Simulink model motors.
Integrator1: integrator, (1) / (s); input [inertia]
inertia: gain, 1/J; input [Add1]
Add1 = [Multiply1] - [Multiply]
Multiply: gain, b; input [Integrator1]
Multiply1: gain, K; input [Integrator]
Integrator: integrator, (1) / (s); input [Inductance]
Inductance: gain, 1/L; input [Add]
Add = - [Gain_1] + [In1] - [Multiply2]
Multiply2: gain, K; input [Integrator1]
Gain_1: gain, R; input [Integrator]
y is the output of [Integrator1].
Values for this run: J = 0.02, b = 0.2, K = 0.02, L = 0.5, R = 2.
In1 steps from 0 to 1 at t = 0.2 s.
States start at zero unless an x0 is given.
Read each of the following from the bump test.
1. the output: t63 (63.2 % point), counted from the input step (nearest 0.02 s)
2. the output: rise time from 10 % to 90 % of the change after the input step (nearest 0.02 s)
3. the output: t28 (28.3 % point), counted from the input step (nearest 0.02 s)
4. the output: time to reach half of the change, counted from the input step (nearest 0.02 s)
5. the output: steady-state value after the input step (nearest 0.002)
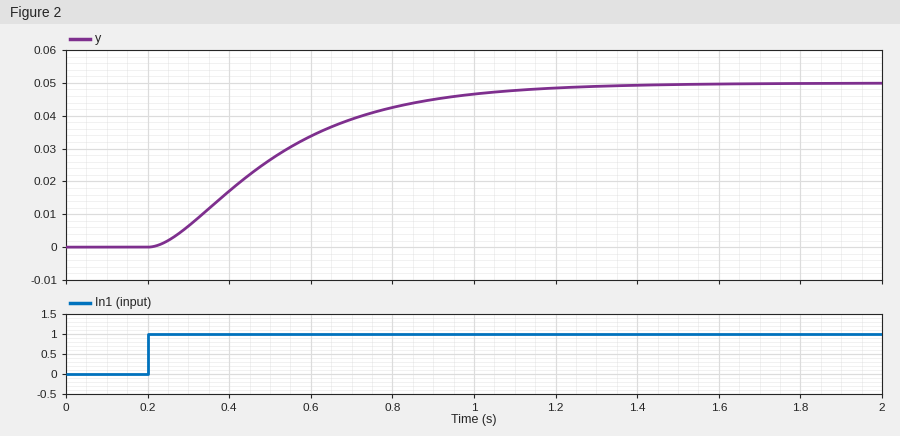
0.36 s
0.62 s
0.18 s
0.28 s
0.050
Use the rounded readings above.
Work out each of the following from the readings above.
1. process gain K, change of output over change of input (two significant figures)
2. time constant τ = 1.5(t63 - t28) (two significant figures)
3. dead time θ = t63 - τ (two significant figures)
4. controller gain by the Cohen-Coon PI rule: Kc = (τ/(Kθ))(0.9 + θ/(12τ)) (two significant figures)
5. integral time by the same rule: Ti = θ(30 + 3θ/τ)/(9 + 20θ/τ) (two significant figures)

0.050
0.27 s
0.090 s
56
0.18 s
